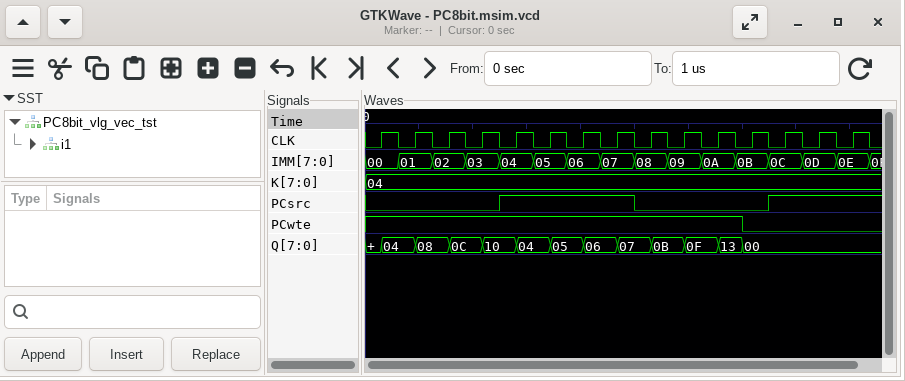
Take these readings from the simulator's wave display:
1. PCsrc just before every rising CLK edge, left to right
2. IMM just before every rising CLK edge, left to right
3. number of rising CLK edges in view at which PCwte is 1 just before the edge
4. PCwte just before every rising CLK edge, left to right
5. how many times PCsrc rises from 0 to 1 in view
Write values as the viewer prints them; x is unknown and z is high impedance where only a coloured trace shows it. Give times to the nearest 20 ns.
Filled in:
0 0 0 0 1 1 1 1 0 0 0 0 1 1 1
00, 01, 02, 03, 04, 05, 06, 07, 08, 09, 0A, 0B, 0C, 0D, 0E
11
1 1 1 1 1 1 1 1 1 1 1 0 0 0 0
2
